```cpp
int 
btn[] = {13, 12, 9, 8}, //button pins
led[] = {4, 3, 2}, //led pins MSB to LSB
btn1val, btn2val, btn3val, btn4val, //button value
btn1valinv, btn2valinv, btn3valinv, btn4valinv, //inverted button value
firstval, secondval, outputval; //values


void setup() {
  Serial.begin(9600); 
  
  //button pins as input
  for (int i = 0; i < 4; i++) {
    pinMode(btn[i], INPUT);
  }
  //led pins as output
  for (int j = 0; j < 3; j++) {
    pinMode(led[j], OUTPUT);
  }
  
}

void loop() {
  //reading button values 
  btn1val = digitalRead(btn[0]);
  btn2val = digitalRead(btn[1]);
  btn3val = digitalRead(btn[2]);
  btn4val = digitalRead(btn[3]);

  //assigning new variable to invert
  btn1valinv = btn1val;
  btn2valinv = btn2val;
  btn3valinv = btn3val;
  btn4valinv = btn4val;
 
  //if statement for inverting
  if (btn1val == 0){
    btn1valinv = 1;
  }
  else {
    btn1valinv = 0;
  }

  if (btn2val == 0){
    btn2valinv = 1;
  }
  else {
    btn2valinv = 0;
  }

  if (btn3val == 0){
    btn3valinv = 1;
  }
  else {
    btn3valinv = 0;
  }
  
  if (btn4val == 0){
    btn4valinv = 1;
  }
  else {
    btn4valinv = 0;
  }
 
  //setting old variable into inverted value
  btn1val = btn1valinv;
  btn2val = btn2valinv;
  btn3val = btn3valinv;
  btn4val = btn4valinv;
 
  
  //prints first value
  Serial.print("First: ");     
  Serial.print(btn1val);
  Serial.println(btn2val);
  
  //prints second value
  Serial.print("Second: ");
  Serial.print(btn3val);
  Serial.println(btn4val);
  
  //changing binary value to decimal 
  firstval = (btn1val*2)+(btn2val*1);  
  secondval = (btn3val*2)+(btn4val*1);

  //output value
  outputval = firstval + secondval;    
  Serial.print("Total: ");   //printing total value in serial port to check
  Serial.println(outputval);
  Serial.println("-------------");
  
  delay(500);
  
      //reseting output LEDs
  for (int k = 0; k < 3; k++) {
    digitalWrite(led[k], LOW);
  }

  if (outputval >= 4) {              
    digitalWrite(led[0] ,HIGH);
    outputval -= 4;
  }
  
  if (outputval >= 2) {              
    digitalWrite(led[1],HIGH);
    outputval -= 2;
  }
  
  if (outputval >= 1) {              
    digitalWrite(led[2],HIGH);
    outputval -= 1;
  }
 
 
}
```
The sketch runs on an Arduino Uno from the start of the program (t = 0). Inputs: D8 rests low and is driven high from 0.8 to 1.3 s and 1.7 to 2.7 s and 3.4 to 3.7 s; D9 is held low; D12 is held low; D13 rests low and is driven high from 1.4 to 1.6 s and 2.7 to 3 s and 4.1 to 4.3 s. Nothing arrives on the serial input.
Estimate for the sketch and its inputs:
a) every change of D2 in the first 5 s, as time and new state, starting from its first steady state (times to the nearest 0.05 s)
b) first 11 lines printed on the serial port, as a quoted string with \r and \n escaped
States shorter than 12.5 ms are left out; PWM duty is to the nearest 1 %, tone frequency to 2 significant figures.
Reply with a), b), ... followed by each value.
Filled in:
a) 0 s low; 1.5 s high; 2 s low; 2.5 s high; 3.5 s low; 4 s high; 4.5 s low
b) "First: 11\r\nSecond: 11\r\nTotal: 6\r\n-------------\r\nFirst: 11\r\nSecond: 11\r\nTotal: 6\r\n-------------\r\nFirst: 11\r\nSecond: 10\r\nTotal: 5\r\n"
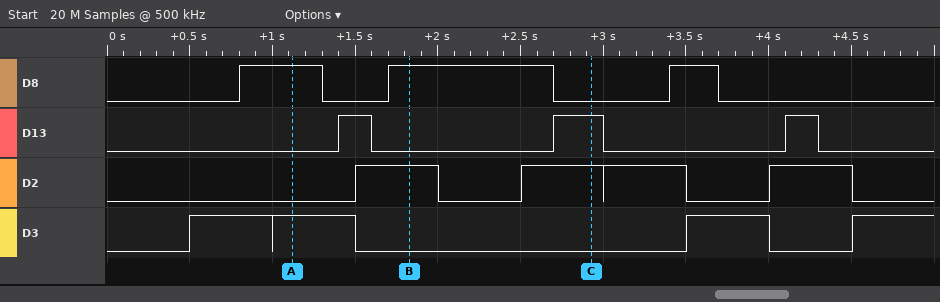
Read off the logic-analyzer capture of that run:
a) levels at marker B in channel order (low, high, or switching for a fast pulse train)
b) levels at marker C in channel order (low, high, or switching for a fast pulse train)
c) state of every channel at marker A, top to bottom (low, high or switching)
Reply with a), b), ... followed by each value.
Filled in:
a) D8 high, D13 low, D2 high, D3 low
b) D8 low, D13 high, D2 high, D3 low
c) D8 high, D13 low, D2 low, D3 high
